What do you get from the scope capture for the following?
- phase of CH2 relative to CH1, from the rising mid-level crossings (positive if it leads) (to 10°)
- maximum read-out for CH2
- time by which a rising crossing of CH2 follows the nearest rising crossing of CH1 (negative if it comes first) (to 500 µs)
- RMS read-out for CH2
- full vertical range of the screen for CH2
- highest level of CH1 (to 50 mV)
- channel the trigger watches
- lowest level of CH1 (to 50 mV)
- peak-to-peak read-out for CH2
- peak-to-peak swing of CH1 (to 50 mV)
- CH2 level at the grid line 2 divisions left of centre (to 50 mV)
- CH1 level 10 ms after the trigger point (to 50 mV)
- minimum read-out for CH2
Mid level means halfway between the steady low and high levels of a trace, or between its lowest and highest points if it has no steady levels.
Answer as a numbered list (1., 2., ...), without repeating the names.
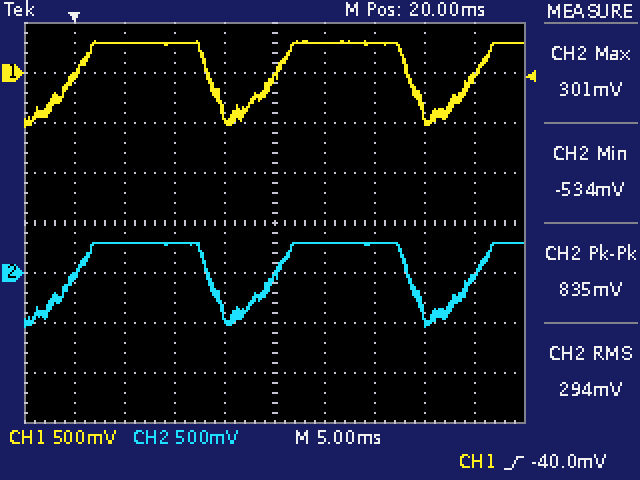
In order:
1. 0°
2. 301 mV
3. 0.0 ms
4. 294 mV
5. 4 V
6. 300 mV
7. CH1
8. -550 mV
9. 835 mV
10. 850 mV
11. 300 mV
12. 300 mV
13. -534 mV
